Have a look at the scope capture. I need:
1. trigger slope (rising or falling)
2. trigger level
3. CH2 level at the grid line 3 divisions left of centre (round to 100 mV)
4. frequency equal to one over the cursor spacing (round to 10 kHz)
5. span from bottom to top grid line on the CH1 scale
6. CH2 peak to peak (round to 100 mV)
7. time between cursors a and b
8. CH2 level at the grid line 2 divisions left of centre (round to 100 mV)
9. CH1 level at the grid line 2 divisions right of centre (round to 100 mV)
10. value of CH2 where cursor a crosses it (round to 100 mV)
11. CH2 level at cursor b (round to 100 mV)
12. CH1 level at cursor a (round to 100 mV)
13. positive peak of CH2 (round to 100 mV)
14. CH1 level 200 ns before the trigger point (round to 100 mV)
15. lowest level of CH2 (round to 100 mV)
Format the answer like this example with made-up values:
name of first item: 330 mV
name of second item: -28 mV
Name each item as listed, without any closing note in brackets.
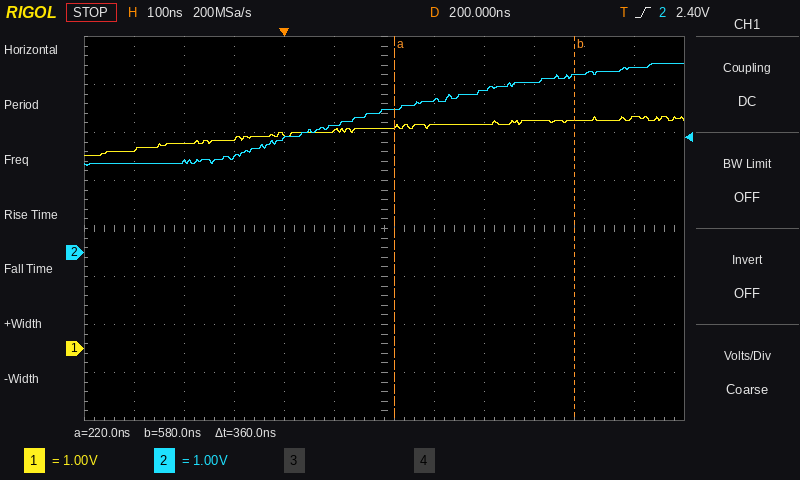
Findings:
trigger slope: rising
trigger level: 2.40 V
CH2 level at the grid line 3 divisions left of centre: 2.0 V
frequency equal to one over the cursor spacing: 2.78 MHz
span from bottom to top grid line on the CH1 scale: 8 V
CH2 peak to peak: 2.1 V
time between cursors a and b: 360 ns
CH2 level at the grid line 2 divisions left of centre: 2.4 V
CH1 level at the grid line 2 divisions right of centre: 4.7 V
value of CH2 where cursor a crosses it: 3.0 V
CH2 level at cursor b: 3.7 V
CH1 level at cursor a: 4.6 V
positive peak of CH2: 3.9 V
CH1 level 200 ns before the trigger point: 4.3 V
lowest level of CH2: 1.8 V
